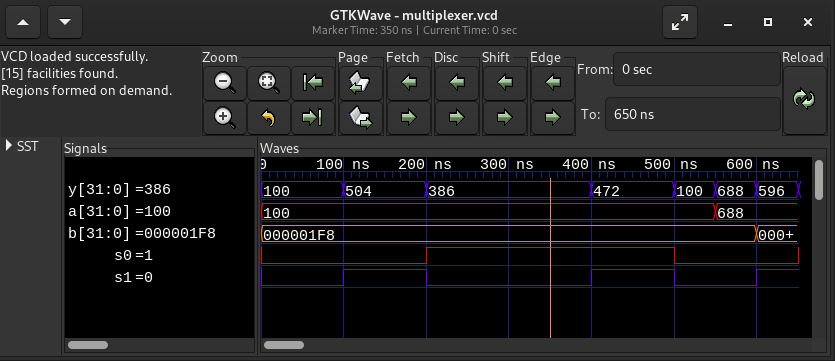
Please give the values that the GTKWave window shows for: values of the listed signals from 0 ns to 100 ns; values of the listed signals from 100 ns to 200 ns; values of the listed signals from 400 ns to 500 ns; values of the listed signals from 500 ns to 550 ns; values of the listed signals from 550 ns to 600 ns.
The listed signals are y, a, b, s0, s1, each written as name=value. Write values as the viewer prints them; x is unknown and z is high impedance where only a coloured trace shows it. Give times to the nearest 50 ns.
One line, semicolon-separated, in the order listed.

y=100, a=100, b=000001F8, s0=0, s1=0; y=504, a=100, b=000001F8, s0=0, s1=1; y=472, a=100, b=000001F8, s0=1, s1=1; y=100, a=100, b=000001F8, s0=0, s1=0; y=688, a=688, b=000001F8, s0=0, s1=0
